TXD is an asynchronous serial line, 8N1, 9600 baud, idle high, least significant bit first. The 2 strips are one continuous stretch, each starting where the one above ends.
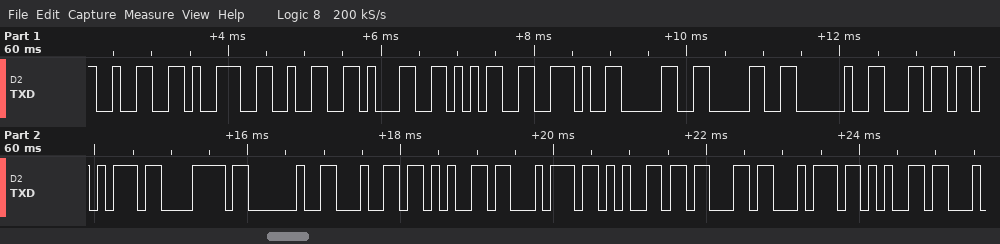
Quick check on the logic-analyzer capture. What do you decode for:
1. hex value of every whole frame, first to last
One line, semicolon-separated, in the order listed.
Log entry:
32 39 32 31 35 2E 30 30 20 6C 75 78 20 64 65 74 65 63 74 65
